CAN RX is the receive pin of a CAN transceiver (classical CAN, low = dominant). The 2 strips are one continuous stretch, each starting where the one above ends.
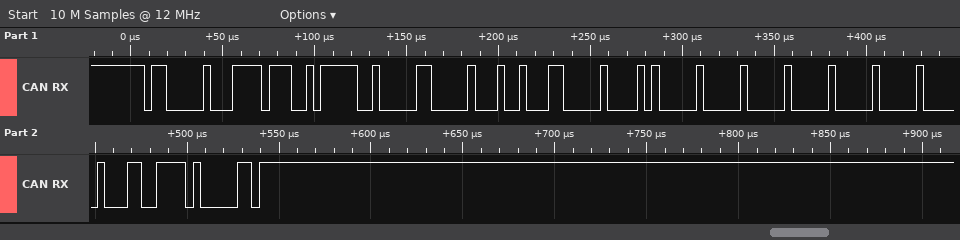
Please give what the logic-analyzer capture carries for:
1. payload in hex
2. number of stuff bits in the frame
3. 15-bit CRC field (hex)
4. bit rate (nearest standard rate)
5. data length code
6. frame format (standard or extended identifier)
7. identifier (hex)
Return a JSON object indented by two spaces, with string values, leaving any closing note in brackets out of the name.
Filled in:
{
  "payload in hex": "04 8C 01 40 00 00 00 00",
  "number of stuff bits in the frame": "13",
  "15-bit CRC field": "0x67A0",
  "bit rate": "250 kbit/s",
  "data length code": "8",
  "frame format": "extended",
  "identifier": "0x1806E5F4"
}
